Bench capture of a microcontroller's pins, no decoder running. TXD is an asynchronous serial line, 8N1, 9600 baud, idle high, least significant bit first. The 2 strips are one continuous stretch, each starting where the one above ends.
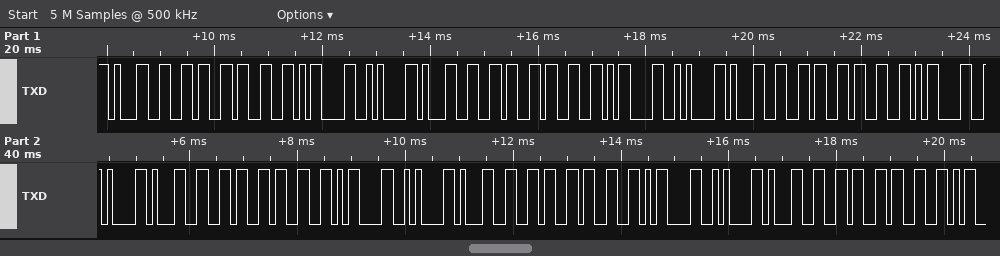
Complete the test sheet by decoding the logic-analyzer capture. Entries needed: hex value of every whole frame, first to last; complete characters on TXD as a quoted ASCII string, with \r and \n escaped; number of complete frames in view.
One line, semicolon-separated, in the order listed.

31 36 33 0D 0A 31 36 33 0D 0A 31 36 33 0D 0A 31 36 33 0D 0A 31 36 33 0D 0A 31 36 33; "163\r\n163\r\n163\r\n163\r\n163\r\n163"; 28
